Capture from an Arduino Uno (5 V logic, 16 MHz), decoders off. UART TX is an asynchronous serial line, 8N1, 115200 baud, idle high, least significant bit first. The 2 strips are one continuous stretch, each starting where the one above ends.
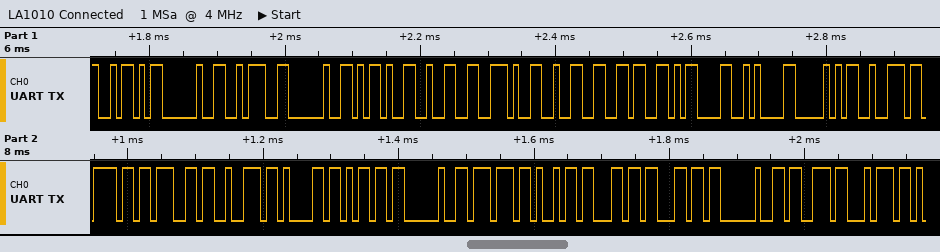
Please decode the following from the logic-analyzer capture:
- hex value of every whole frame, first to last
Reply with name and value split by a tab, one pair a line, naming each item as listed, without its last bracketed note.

hex value of every whole frame, first to last	5A 20 3A 20 2D 32 2E 32 36 0D 0A 50 72 6F 67 72 61 6D 20 77 69 6C 6C 20 73 74
